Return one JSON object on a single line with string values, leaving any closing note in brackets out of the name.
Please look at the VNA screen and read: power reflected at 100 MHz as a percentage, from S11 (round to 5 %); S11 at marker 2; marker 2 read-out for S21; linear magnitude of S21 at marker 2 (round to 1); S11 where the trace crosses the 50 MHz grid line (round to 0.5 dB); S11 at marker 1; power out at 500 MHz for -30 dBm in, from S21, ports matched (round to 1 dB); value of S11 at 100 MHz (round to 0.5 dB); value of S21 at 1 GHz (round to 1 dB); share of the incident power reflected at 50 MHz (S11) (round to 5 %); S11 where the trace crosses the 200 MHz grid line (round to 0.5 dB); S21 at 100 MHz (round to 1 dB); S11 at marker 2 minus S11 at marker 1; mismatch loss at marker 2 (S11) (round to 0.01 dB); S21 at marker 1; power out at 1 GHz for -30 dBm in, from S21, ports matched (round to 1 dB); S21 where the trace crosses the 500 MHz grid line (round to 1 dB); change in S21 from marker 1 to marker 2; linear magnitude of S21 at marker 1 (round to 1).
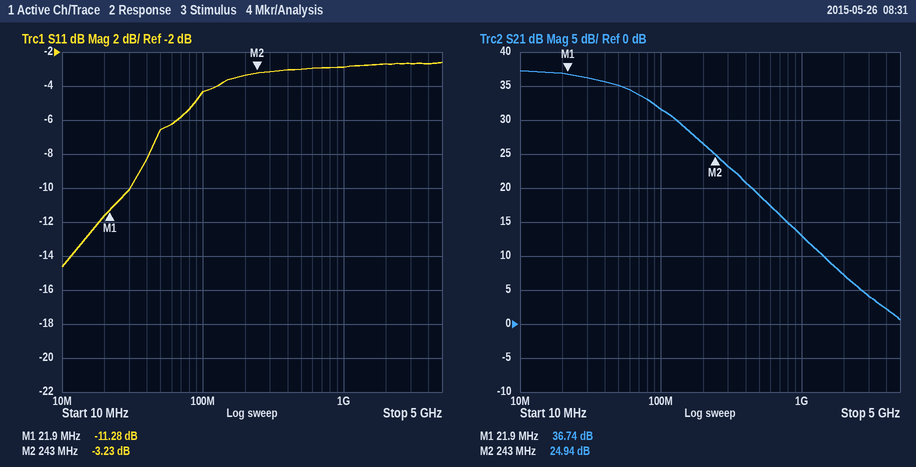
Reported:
{"power reflected at 100 MHz as a percentage, from S11": "35 %", "S11 at marker 2": "-3.23 dB", "marker 2 read-out for S21": "24.94 dB", "linear magnitude of S21 at marker 2": "18", "S11 where the trace crosses the 50 MHz grid line": "-6.5 dB", "S11 at marker 1": "-11.28 dB", "power out at 500 MHz for -30 dBm in, from S21, ports matched": "-11 dBm", "value of S11 at 100 MHz": "-4.5 dB", "value of S21 at 1 GHz": "13 dB", "share of the incident power reflected at 50 MHz (S11)": "20 %", "S11 where the trace crosses the 200 MHz grid line": "-3.5 dB", "S21 at 100 MHz": "32 dB", "S11 at marker 2 minus S11 at marker 1": "8.05 dB", "mismatch loss at marker 2 (S11)": "2.80 dB", "S21 at marker 1": "36.74 dB", "power out at 1 GHz for -30 dBm in, from S21, ports matched": "-17 dBm", "S21 where the trace crosses the 500 MHz grid line": "19 dB", "change in S21 from marker 1 to marker 2": "-11.80 dB", "linear magnitude of S21 at marker 1": "69"}
